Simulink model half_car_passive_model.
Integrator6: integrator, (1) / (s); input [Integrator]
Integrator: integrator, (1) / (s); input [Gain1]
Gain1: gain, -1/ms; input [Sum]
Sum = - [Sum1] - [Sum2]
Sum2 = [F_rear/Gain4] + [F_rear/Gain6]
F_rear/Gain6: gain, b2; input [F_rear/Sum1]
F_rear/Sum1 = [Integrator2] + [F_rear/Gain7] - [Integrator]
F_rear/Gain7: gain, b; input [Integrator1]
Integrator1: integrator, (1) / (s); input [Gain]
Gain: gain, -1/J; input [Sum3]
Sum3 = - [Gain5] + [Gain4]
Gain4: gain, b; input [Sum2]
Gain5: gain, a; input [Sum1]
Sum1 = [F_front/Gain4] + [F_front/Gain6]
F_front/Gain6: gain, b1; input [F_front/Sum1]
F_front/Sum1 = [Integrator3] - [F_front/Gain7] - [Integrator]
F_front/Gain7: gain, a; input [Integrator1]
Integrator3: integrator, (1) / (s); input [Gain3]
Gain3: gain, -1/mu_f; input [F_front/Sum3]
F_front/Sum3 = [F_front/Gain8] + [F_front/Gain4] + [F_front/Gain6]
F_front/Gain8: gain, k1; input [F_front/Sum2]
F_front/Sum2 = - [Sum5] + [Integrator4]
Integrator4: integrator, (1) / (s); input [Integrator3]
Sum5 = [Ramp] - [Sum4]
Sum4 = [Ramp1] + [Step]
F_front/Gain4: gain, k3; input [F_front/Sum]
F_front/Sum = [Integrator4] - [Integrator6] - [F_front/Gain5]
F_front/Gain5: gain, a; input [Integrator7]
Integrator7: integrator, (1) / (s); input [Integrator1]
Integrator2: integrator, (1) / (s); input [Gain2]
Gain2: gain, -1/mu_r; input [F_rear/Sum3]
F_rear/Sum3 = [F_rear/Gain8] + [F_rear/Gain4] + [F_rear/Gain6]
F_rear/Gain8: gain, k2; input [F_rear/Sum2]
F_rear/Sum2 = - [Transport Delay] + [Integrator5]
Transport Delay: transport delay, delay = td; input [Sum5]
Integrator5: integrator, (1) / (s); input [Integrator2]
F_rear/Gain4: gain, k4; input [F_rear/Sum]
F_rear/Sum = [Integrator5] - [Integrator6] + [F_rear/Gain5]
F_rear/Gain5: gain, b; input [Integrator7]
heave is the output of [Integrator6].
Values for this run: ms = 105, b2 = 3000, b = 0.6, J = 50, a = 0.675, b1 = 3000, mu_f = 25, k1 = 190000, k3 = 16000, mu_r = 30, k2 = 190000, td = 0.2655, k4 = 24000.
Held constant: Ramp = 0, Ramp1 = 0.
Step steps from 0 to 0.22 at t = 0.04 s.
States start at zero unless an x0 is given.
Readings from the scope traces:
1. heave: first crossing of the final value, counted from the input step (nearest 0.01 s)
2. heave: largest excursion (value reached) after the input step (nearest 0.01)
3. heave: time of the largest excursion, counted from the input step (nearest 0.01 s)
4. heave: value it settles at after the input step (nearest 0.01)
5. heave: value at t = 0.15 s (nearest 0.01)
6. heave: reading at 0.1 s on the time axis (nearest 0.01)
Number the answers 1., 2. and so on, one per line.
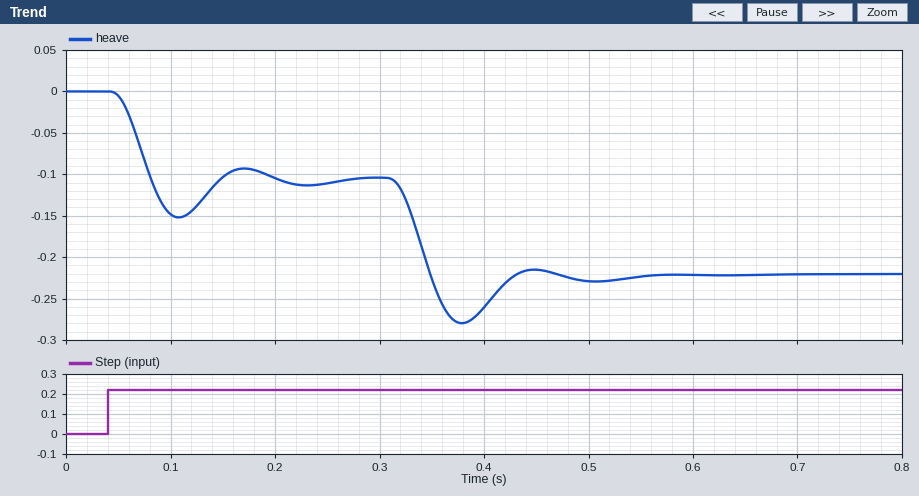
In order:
1. 0.31 s
2. -0.28
3. 0.34 s
4. -0.22
5. -0.10
6. -0.15
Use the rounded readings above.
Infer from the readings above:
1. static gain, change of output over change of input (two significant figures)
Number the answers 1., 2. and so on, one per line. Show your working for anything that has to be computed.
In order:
1. (-0.22 - 0) / (0.22 - 0) = -1.0
